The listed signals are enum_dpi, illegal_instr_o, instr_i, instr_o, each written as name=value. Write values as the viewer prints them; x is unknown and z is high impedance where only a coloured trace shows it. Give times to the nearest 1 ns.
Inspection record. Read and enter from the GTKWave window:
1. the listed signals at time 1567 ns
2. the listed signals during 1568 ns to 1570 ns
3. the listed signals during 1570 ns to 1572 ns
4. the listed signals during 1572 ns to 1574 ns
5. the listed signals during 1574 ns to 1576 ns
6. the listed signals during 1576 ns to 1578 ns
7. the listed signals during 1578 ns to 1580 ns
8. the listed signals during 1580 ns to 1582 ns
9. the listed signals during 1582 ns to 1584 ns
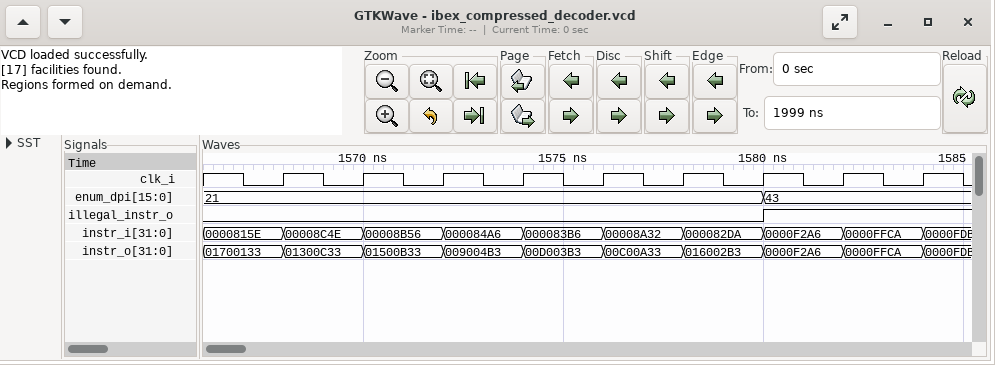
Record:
enum_dpi=21, illegal_instr_o=0, instr_i=0000815E, instr_o=01700133
enum_dpi=21, illegal_instr_o=0, instr_i=00008C4E, instr_o=01300C33
enum_dpi=21, illegal_instr_o=0, instr_i=00008B56, instr_o=01500B33
enum_dpi=21, illegal_instr_o=0, instr_i=000084A6, instr_o=009004B3
enum_dpi=21, illegal_instr_o=0, instr_i=000083B6, instr_o=00D003B3
enum_dpi=21, illegal_instr_o=0, instr_i=00008A32, instr_o=00C00A33
enum_dpi=21, illegal_instr_o=0, instr_i=000082DA, instr_o=016002B3
enum_dpi=43, illegal_instr_o=1, instr_i=0000F2A6, instr_o=0000F2A6
enum_dpi=43, illegal_instr_o=1, instr_i=0000FFCA, instr_o=0000FFCA
